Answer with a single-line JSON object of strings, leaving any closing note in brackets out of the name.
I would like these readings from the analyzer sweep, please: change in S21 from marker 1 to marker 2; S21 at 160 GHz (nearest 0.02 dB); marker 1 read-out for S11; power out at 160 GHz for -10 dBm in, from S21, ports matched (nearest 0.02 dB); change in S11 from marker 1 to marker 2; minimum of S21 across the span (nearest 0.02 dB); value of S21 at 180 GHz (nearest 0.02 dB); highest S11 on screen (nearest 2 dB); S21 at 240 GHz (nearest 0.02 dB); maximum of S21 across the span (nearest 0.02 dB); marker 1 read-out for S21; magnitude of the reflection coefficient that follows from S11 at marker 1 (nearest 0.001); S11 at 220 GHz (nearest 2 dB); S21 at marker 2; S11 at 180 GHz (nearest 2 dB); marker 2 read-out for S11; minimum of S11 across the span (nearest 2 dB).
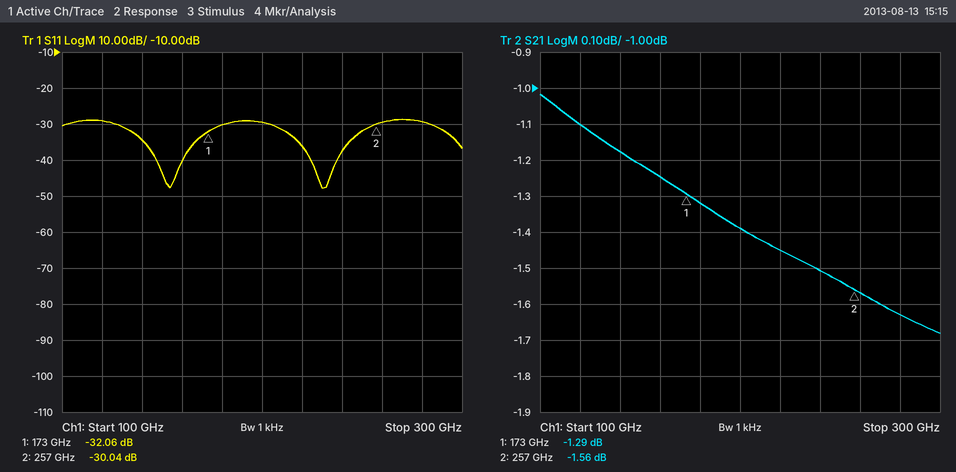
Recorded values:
{"change in S21 from marker 1 to marker 2": "-0.27 dB", "S21 at 160 GHz": "-1.24 dB", "marker 1 read-out for S11": "-32.06 dB", "power out at 160 GHz for -10 dBm in, from S21, ports matched": "-11.24 dBm", "change in S11 from marker 1 to marker 2": "2.02 dB", "minimum of S21 across the span": "-1.68 dB", "value of S21 at 180 GHz": "-1.32 dB", "highest S11 on screen": "-28 dB", "S21 at 240 GHz": "-1.50 dB", "maximum of S21 across the span": "-1.02 dB", "marker 1 read-out for S21": "-1.29 dB", "magnitude of the reflection coefficient that follows from S11 at marker 1": "0.025", "S11 at 220 GHz": "-36 dB", "S21 at marker 2": "-1.56 dB", "S11 at 180 GHz": "-30 dB", "marker 2 read-out for S11": "-30.04 dB", "minimum of S11 across the span": "-48 dB"}
